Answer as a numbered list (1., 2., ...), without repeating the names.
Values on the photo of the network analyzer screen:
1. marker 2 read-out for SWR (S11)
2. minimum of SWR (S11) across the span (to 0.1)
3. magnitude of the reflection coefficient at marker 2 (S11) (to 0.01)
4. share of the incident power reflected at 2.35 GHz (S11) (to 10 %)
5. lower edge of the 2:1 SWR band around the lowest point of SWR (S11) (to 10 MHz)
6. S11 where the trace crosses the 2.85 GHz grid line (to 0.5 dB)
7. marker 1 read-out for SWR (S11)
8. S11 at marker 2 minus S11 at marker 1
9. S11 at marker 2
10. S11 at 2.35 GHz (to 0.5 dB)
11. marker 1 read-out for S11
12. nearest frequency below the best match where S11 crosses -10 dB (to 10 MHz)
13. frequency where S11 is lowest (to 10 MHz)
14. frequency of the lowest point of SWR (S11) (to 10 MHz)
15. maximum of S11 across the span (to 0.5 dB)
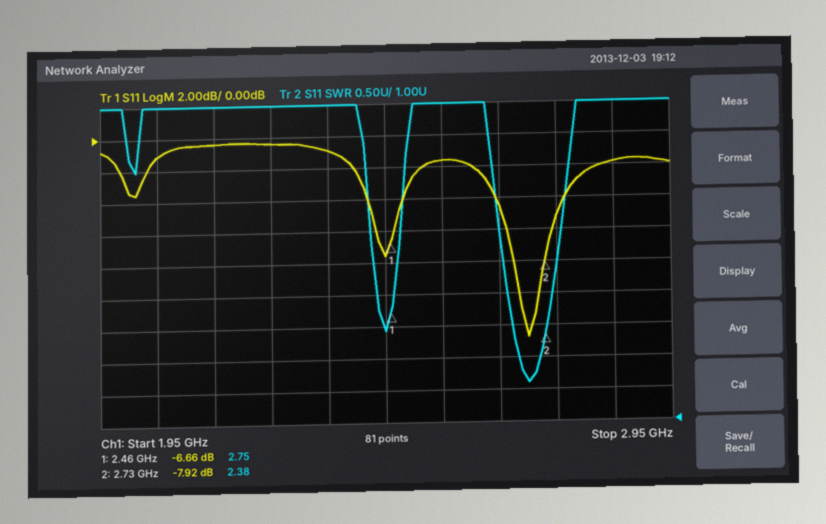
1. 2.38
2. 1.6
3. 0.40
4. 80 %
5. 2.68 GHz
6. -2.0 dB
7. 2.75
8. -1.26 dB
9. -7.92 dB
10. -1.0 dB
11. -6.66 dB
12. 2.68 GHz
13. 2.70 GHz
14. 2.70 GHz
15. -0.5 dB
